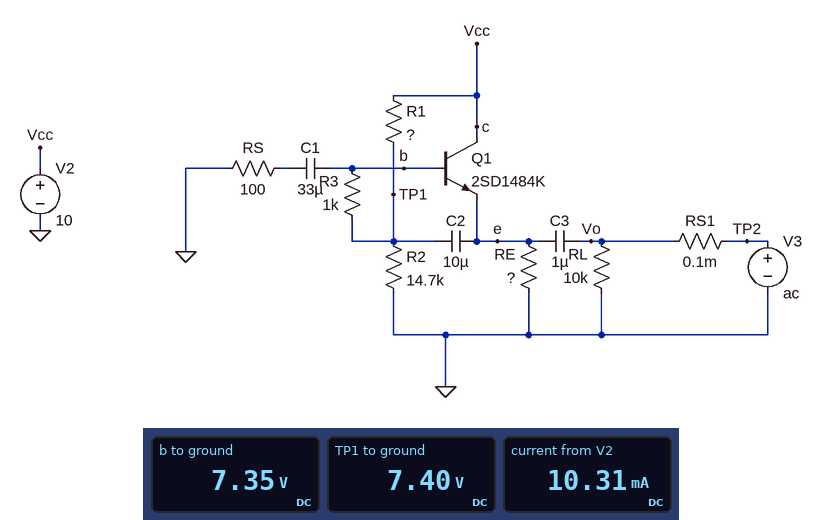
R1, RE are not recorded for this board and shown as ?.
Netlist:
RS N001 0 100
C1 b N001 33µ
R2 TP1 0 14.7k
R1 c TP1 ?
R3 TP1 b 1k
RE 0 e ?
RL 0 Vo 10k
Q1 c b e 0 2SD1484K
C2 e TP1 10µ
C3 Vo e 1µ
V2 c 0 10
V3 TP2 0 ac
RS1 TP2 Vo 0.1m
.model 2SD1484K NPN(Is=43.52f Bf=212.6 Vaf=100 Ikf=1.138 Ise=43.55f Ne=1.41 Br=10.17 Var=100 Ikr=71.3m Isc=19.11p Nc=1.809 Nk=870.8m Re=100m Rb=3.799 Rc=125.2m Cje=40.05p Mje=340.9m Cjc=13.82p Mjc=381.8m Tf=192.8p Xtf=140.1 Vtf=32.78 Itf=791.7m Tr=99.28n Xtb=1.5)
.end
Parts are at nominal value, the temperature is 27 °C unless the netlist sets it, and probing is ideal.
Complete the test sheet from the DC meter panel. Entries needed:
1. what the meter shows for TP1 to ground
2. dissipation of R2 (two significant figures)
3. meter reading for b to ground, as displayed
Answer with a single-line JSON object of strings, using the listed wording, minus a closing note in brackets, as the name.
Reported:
{"what the meter shows for TP1 to ground": "7.40 V", "dissipation of R2": "3.7 mW", "meter reading for b to ground, as displayed": "7.35 V"}
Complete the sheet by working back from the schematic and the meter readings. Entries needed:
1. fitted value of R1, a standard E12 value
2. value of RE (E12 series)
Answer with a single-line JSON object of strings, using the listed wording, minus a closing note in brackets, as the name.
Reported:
{"fitted value of R1, a standard E12 value": "4.7 kΩ", "value of RE": "680 Ω"}
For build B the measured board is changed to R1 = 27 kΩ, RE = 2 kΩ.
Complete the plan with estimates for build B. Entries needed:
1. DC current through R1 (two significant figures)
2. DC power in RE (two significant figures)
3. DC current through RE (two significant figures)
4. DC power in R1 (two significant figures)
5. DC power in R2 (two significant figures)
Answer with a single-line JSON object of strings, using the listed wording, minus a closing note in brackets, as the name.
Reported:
{"DC current through R1": "240 µA", "DC power in RE": "4.0 mW", "DC current through RE": "1.4 mA", "DC power in R1": "1.6 mW", "DC power in R2": "810 µW"}
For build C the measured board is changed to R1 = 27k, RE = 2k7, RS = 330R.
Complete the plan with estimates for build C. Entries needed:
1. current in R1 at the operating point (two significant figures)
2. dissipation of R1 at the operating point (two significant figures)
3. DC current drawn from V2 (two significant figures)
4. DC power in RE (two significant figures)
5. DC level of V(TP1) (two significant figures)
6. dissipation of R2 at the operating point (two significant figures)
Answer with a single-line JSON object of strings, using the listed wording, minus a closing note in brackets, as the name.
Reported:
{"current in R1 at the operating point": "240 µA", "dissipation of R1 at the operating point": "1.6 mW", "DC current drawn from V2": "1.3 mA", "DC power in RE": "3.0 mW", "DC level of V(TP1)": "3.5 V", "dissipation of R2 at the operating point": "820 µW"}
